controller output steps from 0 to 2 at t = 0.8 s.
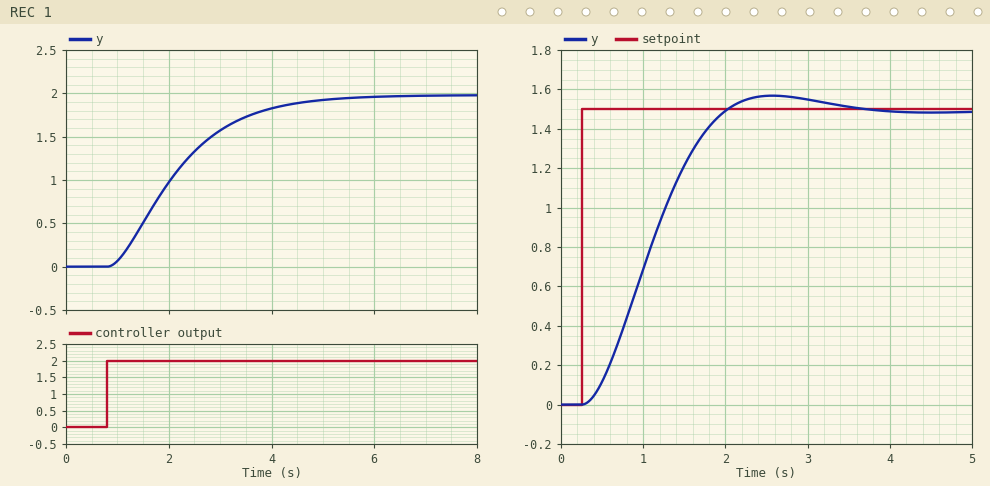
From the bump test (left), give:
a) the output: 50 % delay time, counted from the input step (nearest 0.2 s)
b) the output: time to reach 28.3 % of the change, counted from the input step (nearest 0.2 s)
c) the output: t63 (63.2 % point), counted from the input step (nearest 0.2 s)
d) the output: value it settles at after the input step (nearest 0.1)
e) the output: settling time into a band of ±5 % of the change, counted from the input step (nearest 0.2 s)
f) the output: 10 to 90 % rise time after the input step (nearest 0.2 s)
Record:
1.2 s
0.8 s
1.6 s
2.0
3.6 s
2.6 s
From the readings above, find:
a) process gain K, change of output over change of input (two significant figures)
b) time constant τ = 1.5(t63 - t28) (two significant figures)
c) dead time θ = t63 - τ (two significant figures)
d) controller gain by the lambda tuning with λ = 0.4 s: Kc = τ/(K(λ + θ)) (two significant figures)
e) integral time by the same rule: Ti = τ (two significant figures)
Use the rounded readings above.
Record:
1.0
1.2 s
0.40 s
1.5
1.2 s
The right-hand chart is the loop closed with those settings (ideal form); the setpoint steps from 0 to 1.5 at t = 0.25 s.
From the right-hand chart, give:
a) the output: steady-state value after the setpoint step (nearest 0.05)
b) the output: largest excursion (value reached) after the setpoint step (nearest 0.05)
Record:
1.50
1.55
